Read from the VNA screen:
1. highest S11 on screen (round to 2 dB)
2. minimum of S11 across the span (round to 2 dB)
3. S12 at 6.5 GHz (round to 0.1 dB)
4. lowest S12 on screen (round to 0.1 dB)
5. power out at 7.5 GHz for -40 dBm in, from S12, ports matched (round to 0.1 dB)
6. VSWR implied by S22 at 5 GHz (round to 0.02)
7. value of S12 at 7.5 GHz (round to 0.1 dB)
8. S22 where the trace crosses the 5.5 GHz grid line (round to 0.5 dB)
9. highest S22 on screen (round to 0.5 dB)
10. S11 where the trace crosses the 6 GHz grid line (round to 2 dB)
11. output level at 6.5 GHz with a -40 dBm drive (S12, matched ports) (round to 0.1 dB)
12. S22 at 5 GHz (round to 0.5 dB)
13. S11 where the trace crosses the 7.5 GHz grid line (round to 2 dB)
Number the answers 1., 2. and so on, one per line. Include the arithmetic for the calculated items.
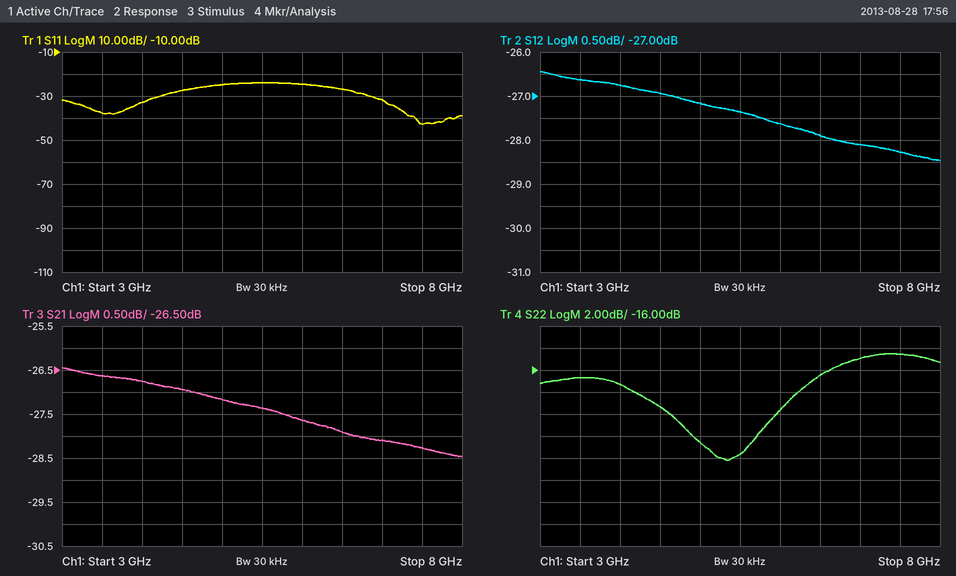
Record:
1. -24 dB
2. -42 dB
3. -27.9 dB
4. -28.5 dB
5. -40 dBm + (-28.3 dB) = -68.3 dBm
6. |Γ| = 10^(-22.5/20) = 0.0750; VSWR = (1 + 0.0750)/(1 − 0.0750) ≈ 1.16
7. -28.3 dB
8. -23.5 dB
9. -14.5 dB
10. -24 dB
11. -40 dBm + (-27.9 dB) = -67.9 dBm
12. -22.5 dB
13. -42 dB
